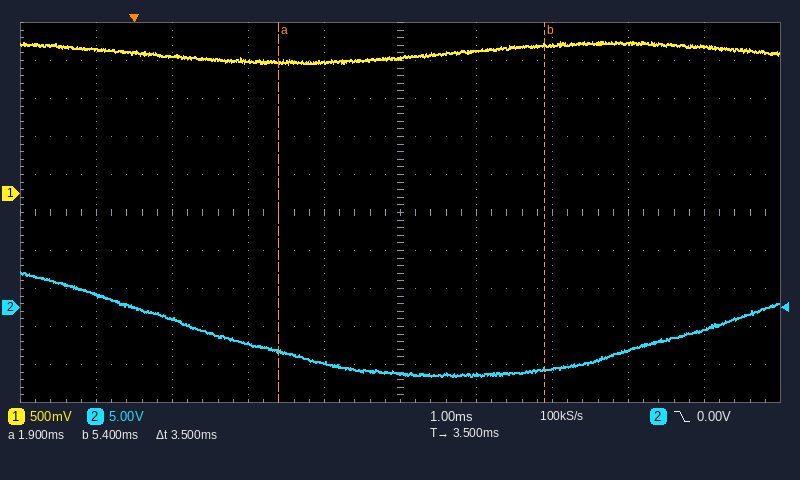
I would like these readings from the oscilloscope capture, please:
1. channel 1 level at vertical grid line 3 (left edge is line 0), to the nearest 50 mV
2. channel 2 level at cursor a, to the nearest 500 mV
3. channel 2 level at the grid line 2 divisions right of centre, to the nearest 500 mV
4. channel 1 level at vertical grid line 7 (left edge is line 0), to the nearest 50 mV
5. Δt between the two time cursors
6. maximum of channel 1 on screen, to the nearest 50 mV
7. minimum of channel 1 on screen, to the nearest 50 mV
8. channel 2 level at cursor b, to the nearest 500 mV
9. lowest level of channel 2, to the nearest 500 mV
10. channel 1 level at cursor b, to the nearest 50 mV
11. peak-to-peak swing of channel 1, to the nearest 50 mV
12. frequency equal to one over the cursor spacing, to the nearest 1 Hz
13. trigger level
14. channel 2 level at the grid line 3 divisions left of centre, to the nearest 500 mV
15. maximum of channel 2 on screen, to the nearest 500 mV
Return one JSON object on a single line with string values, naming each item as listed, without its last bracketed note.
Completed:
{"channel 1 level at vertical grid line 3 (left edge is line 0), to the nearest 50 mV": "1.75 V", "channel 2 level at cursor a, to the nearest 500 mV": "-5.5 V", "channel 2 level at the grid line 2 divisions right of centre, to the nearest 500 mV": "-8.0 V", "channel 1 level at vertical grid line 7 (left edge is line 0), to the nearest 50 mV": "1.95 V", "Δt between the two time cursors": "3.5 ms", "maximum of channel 1 on screen, to the nearest 50 mV": "2.00 V", "minimum of channel 1 on screen, to the nearest 50 mV": "1.70 V", "channel 2 level at cursor b, to the nearest 500 mV": "-8.0 V", "lowest level of channel 2, to the nearest 500 mV": "-9.0 V", "channel 1 level at cursor b, to the nearest 50 mV": "1.95 V", "peak-to-peak swing of channel 1, to the nearest 50 mV": "300 mV", "frequency equal to one over the cursor spacing, to the nearest 1 Hz": "286 Hz", "trigger level": "0.00 V", "channel 2 level at the grid line 3 divisions left of centre, to the nearest 500 mV": "-1.5 V", "maximum of channel 2 on screen, to the nearest 500 mV": "4.5 V"}
